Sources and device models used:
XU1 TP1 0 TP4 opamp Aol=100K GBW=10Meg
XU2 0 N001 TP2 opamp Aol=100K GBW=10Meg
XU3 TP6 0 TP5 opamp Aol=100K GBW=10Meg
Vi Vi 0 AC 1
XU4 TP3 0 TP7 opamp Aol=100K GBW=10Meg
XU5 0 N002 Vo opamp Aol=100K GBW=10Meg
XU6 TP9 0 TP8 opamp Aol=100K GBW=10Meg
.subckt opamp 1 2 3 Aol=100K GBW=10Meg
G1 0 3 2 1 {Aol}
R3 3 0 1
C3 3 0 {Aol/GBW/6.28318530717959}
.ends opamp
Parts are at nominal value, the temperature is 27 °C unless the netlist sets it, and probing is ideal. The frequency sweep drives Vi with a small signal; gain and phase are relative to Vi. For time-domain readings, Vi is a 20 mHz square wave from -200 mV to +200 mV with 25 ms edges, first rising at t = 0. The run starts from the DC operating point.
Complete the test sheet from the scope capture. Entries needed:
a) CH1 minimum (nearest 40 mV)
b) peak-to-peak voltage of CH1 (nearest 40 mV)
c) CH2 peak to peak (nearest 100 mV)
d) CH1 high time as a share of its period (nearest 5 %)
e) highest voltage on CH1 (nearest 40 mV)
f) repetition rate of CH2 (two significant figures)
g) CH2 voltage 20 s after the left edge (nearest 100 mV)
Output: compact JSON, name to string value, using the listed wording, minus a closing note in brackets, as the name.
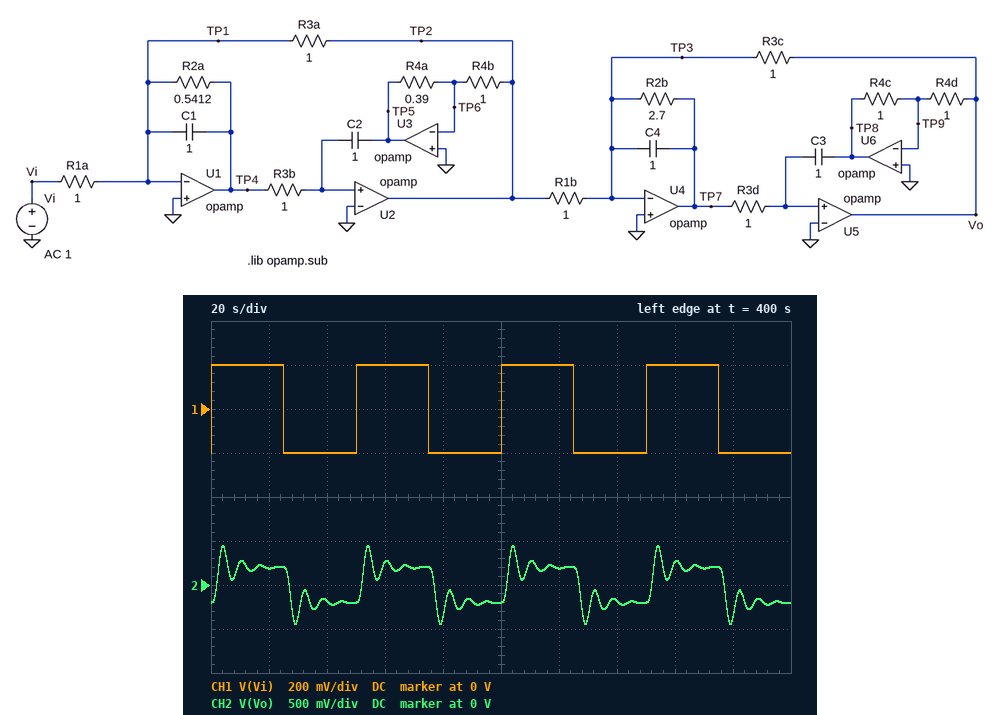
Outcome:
{"CH1 minimum": "-200 mV", "peak-to-peak voltage of CH1": "400 mV", "CH2 peak to peak": "900 mV", "CH1 high time as a share of its period": "50 %", "highest voltage on CH1": "200 mV", "repetition rate of CH2": "20 mHz", "CH2 voltage 20 s after the left edge": "200 mV"}
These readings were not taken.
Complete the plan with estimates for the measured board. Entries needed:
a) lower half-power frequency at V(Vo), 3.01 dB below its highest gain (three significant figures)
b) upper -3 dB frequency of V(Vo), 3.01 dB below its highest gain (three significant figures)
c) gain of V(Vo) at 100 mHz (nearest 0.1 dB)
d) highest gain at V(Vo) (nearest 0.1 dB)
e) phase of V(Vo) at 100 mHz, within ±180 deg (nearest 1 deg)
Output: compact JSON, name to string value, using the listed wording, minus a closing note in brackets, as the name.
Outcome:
{"lower half-power frequency at V(Vo), 3.01 dB below its highest gain": "120 mHz", "upper -3 dB frequency of V(Vo), 3.01 dB below its highest gain": "180 mHz", "gain of V(Vo) at 100 mHz": "4.1 dB", "highest gain at V(Vo)": "9.3 dB", "phase of V(Vo) at 100 mHz, within ±180 deg": "-49 deg"}
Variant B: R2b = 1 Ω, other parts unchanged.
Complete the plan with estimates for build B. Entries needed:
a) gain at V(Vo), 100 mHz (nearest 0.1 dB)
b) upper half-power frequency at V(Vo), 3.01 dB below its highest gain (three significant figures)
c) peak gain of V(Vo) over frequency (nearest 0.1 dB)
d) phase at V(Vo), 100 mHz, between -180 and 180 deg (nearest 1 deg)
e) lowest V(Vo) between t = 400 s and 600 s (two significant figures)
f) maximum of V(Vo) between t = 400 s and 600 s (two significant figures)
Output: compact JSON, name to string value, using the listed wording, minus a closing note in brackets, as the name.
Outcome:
{"gain at V(Vo), 100 mHz": "1.5 dB", "upper half-power frequency at V(Vo), 3.01 dB below its highest gain": "185 mHz", "peak gain of V(Vo) over frequency": "1.7 dB", "phase at V(Vo), 100 mHz, between -180 and 180 deg": "-74 deg", "lowest V(Vo) between t = 400 s and 600 s": "-290 mV", "maximum of V(Vo) between t = 400 s and 600 s": "290 mV"}
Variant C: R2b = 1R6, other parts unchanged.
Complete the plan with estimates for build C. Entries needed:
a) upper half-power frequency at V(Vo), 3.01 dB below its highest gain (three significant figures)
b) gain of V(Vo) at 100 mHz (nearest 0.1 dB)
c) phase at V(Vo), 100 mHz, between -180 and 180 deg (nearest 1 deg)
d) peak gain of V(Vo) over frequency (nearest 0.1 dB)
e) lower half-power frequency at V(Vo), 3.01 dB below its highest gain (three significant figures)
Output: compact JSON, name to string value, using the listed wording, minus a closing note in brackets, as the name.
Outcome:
{"upper half-power frequency at V(Vo), 3.01 dB below its highest gain": "186 mHz", "gain of V(Vo) at 100 mHz": "3.2 dB", "phase at V(Vo), 100 mHz, between -180 and 180 deg": "-61 deg", "peak gain of V(Vo) over frequency": "5.0 dB", "lower half-power frequency at V(Vo), 3.01 dB below its highest gain": "79.1 mHz"}
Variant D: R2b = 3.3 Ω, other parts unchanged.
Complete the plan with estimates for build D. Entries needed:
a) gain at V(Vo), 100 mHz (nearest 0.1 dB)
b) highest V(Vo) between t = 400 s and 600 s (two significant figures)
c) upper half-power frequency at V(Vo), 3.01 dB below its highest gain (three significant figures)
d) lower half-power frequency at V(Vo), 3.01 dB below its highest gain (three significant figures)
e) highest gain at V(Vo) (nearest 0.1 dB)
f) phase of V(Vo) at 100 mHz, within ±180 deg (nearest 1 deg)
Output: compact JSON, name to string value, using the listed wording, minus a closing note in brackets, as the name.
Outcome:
{"gain at V(Vo), 100 mHz": "4.3 dB", "highest V(Vo) between t = 400 s and 600 s": "460 mV", "upper half-power frequency at V(Vo), 3.01 dB below its highest gain": "178 mHz", "lower half-power frequency at V(Vo), 3.01 dB below its highest gain": "129 mHz", "highest gain at V(Vo)": "11.0 dB", "phase of V(Vo) at 100 mHz, within ±180 deg": "-46 deg"}
